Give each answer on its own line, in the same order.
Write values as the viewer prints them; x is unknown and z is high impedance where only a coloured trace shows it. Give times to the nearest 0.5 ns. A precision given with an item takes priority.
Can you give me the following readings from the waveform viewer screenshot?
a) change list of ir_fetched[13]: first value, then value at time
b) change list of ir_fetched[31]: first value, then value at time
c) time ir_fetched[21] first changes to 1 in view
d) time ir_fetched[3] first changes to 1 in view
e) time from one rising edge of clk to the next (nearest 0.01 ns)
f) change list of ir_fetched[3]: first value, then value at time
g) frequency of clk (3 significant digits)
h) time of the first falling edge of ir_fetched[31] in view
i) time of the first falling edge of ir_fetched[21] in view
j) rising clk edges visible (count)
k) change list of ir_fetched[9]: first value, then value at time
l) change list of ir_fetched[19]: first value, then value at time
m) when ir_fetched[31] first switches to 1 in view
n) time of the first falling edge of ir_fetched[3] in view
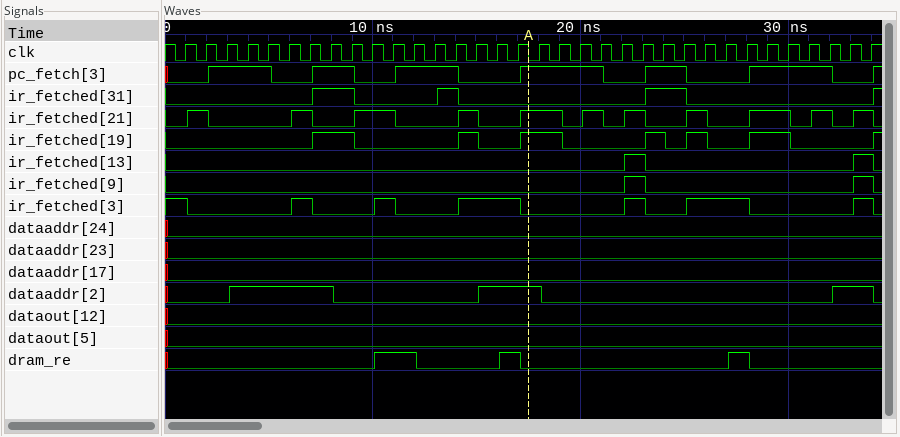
0, 1 at 22 ns, 0 at 23 ns, 1 at 33 ns, 0 at 34 ns
0, 1 at 7 ns, 0 at 9 ns, 1 at 13 ns, 0 at 14 ns, 1 at 23 ns, 0 at 25 ns, 1 at 34 ns
1 ns
6 ns
1 ns
1, 0 at 1 ns, 1 at 6 ns, 0 at 7 ns, 1 at 10 ns, 0 at 11 ns, 1 at 14 ns, 0 at 17 ns, 1 at 22 ns, 0 at 23 ns, 1 at 25 ns, 0 at 28 ns, 1 at 33 ns, 0 at 34 ns
1.00 GHz
9 ns
2 ns
34
0, 1 at 22 ns, 0 at 23 ns, 1 at 33 ns, 0 at 34 ns
0, 1 at 7 ns, 0 at 9 ns, 1 at 14 ns, 0 at 15 ns, 1 at 17 ns, 0 at 19 ns, 1 at 23 ns, 0 at 24 ns, 1 at 25 ns, 0 at 26 ns, 1 at 28 ns, 0 at 30 ns, 1 at 34 ns
7 ns
1 ns
